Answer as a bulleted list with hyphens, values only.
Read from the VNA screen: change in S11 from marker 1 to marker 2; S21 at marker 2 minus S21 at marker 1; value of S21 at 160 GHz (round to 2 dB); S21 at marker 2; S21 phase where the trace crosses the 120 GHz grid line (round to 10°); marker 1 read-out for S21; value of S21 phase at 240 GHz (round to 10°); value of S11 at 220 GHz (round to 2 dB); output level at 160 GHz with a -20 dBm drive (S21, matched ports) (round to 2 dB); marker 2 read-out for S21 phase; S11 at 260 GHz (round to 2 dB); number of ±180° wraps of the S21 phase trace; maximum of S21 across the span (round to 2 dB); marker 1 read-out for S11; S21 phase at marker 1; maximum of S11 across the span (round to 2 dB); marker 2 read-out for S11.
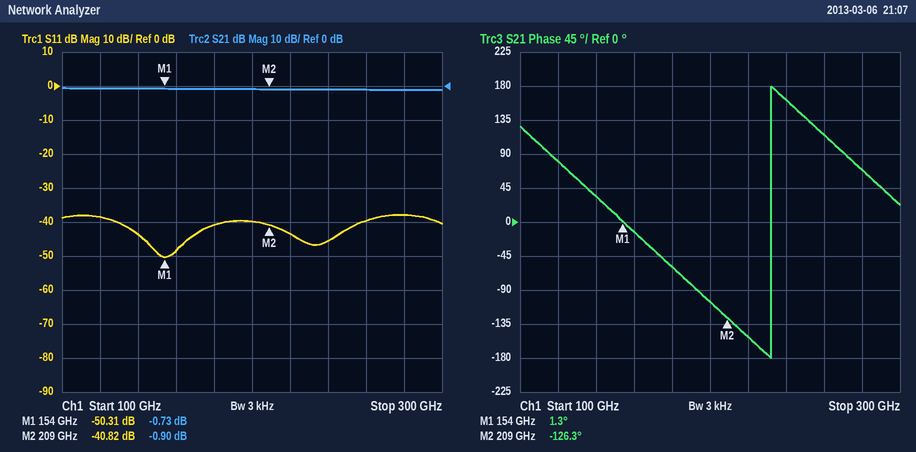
- 9.49 dB
- -0.17 dB
- 0 dB
- -0.90 dB
- 80°
- -0.73 dB
- 160°
- -44 dB
- -20 dBm
- -126.3°
- -40 dB
- 1
- 0 dB
- -50.31 dB
- 1.3°
- -38 dB
- -40.82 dB
